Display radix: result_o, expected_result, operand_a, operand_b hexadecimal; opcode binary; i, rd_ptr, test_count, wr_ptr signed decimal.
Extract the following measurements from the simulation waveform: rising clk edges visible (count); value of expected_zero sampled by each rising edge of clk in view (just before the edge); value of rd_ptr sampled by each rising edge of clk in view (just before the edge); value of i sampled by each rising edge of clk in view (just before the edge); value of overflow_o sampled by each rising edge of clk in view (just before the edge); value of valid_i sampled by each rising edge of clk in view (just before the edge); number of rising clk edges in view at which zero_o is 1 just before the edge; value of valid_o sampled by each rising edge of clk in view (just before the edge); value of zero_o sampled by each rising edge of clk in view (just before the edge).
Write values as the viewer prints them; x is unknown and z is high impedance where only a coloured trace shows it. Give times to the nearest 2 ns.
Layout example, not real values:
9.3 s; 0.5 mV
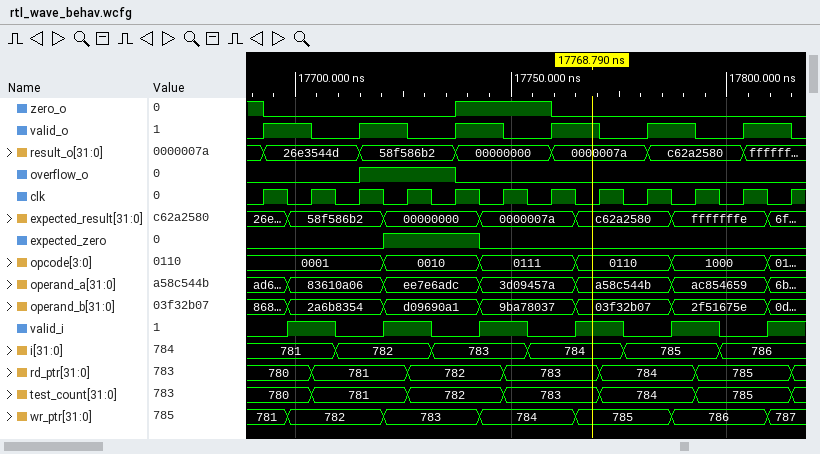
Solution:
12; 0 0 0 1 1 0 0 0 0 0 0 0; 780, 780, 781, 781, 782, 782, 783, 783, 784, 784, 785, 785; 781, 781, 782, 782, 783, 783, 784, 784, 785, 785, 786, 786; 0 0 0 1 1 0 0 0 0 0 0 0; 0 1 0 1 0 1 0 1 0 1 0 1; 3; 0 1 0 1 0 1 0 1 0 1 0 1; 1 0 0 0 0 1 1 0 0 0 0 0
